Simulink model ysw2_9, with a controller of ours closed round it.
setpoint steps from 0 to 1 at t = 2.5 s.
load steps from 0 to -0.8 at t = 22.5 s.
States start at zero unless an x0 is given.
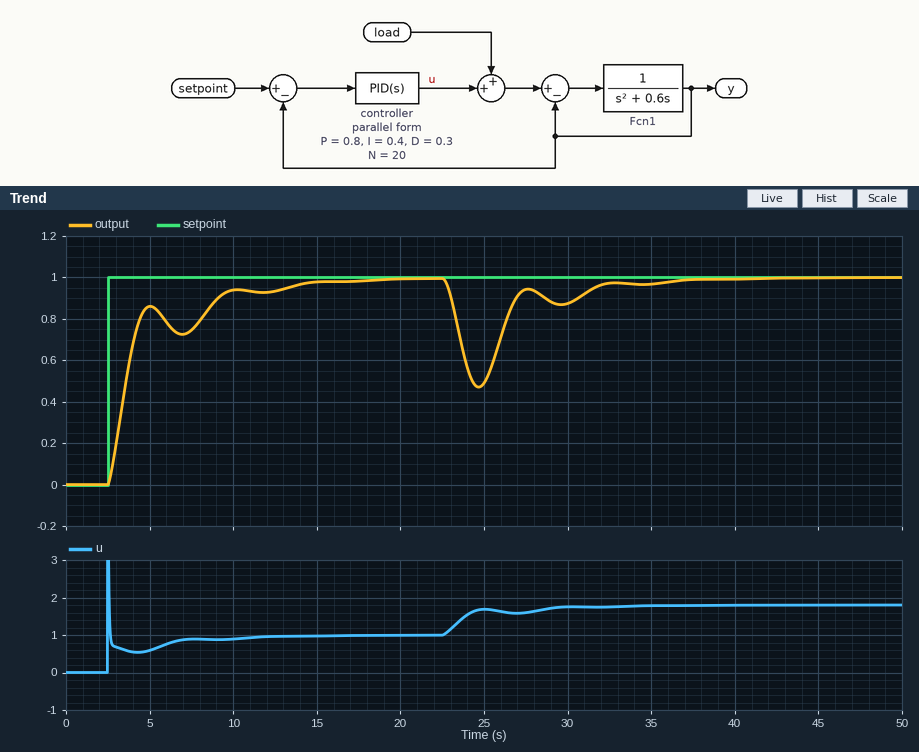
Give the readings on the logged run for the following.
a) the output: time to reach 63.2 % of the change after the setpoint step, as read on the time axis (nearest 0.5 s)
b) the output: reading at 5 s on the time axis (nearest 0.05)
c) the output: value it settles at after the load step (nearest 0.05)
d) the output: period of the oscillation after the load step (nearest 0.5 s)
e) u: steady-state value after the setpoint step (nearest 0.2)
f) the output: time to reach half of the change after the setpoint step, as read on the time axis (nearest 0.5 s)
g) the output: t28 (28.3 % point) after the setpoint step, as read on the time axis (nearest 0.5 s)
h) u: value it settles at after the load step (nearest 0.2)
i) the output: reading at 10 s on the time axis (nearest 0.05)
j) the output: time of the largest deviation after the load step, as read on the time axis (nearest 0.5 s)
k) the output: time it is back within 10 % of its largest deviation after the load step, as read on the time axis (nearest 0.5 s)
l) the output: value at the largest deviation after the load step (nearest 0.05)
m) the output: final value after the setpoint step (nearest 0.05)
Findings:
4.0 s
0.85
1.00
5.0 s
1.0
3.5 s
3.0 s
1.8
0.95
24.5 s
31.5 s
0.45
1.00
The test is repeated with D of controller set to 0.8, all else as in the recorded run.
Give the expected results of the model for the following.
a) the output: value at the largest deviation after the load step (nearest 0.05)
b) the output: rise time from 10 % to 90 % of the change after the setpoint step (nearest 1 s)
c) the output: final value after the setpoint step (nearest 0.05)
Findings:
0.55
7 s
1.00
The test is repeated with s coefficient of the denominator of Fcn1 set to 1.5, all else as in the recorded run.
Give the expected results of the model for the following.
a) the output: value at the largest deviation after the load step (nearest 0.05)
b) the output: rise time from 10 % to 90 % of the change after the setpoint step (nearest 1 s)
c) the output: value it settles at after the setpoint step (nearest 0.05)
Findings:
0.60
6 s
1.00
